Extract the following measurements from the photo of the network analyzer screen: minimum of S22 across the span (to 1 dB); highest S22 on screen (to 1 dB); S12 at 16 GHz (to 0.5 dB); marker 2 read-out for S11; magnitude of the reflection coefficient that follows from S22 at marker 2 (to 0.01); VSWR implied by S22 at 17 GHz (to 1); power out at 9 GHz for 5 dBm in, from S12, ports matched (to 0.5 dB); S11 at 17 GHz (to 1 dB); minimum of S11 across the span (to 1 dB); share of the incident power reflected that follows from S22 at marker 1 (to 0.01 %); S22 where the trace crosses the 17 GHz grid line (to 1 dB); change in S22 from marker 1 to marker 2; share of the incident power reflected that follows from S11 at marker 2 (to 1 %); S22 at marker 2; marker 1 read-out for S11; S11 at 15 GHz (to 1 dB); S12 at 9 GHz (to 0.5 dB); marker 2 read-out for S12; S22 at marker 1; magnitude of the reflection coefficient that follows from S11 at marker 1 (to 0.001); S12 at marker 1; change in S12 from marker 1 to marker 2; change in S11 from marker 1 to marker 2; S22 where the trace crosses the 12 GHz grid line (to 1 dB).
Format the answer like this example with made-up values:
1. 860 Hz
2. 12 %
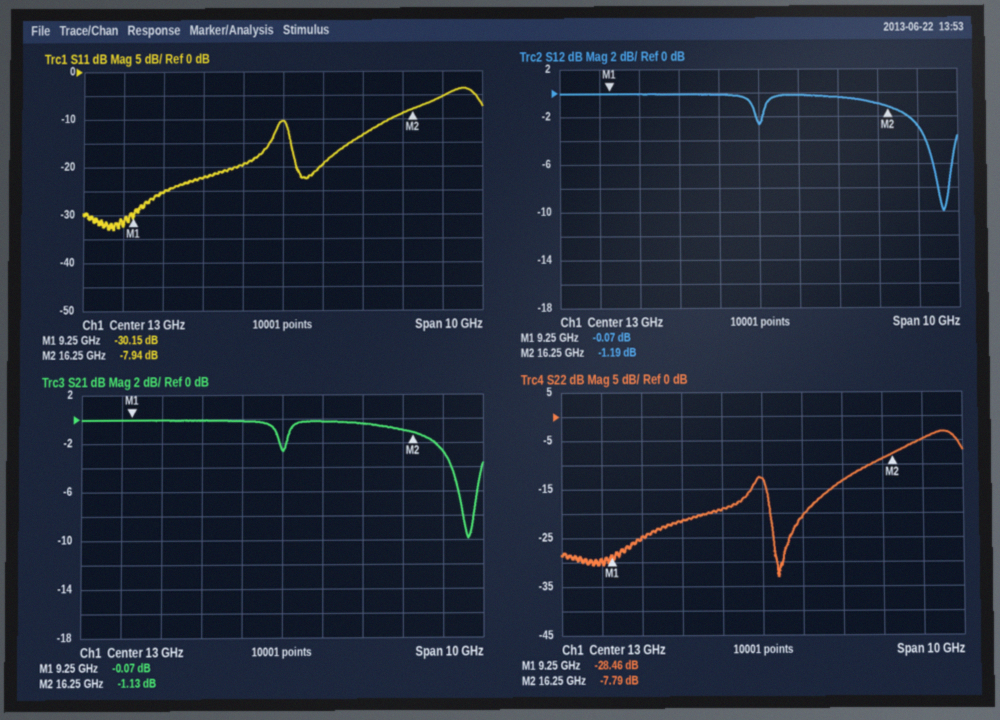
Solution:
1. -33 dB
2. -3 dB
3. -1.0 dB
4. -7.94 dB
5. 0.41
6. 4
7. 5.0 dBm
8. -5 dB
9. -33 dB
10. 0.14 %
11. -5 dB
12. 20.67 dB
13. 16 %
14. -7.79 dB
15. -30.15 dB
16. -13 dB
17. 0.0 dB
18. -1.19 dB
19. -28.46 dB
20. 0.031
21. -0.07 dB
22. -1.12 dB
23. 22.21 dB
24. -19 dB
